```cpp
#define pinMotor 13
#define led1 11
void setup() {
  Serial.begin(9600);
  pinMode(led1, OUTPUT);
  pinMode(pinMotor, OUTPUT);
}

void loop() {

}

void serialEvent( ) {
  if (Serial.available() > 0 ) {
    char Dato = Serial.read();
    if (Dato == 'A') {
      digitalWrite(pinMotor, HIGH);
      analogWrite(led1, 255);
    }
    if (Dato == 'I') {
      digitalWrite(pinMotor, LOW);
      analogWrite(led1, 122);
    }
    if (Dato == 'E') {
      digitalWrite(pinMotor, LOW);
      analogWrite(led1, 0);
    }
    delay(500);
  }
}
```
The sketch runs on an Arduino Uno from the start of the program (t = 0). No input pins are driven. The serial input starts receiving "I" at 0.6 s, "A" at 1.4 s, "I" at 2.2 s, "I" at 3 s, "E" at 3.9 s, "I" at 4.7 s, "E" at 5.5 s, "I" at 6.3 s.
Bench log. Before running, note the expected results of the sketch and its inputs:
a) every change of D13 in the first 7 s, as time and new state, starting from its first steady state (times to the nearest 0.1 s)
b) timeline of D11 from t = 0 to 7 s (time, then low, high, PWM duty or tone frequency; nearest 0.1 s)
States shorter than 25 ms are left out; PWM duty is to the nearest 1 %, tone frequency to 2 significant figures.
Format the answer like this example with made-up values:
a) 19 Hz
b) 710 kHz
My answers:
a) 0 s low; 1.4 s high; 2.2 s low
b) 0 s low; 0.6 s PWM 48 %; 1.4 s high; 2.2 s PWM 48 %; 3.9 s low; 4.7 s PWM 48 %; 5.5 s low; 6.3 s PWM 48 %
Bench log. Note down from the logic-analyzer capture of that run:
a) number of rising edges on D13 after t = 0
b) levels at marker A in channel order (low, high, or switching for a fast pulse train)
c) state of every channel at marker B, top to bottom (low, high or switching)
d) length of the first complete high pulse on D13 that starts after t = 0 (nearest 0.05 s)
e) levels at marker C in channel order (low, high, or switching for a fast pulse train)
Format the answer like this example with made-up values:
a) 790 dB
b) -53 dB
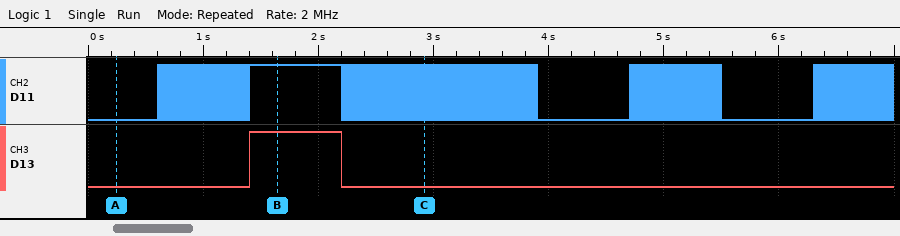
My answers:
a) 1
b) D11 low, D13 low
c) D11 high, D13 high
d) 0.80 s
e) D11 switching, D13 low
